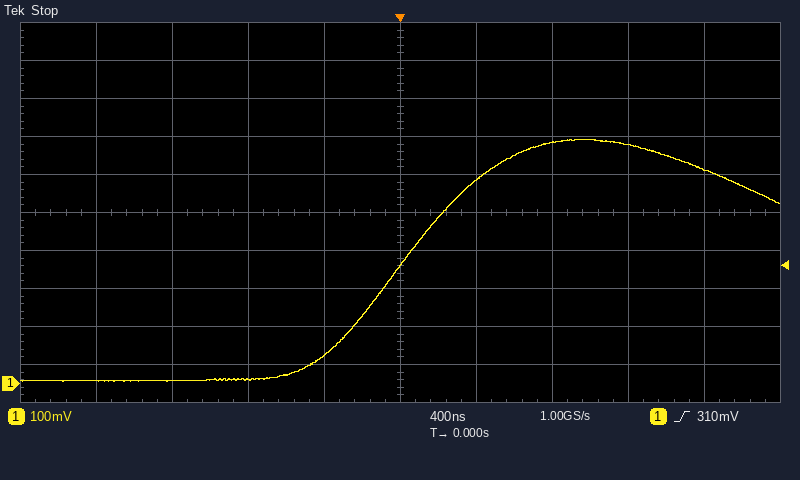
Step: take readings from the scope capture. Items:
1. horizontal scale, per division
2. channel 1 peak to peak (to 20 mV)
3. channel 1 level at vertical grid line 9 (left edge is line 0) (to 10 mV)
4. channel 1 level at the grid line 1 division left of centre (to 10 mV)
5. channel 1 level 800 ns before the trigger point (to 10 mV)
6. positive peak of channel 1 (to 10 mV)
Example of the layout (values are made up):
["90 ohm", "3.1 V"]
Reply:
["400 ns", "640 mV", "560 mV", "70 mV", "10 mV", "640 mV"]
